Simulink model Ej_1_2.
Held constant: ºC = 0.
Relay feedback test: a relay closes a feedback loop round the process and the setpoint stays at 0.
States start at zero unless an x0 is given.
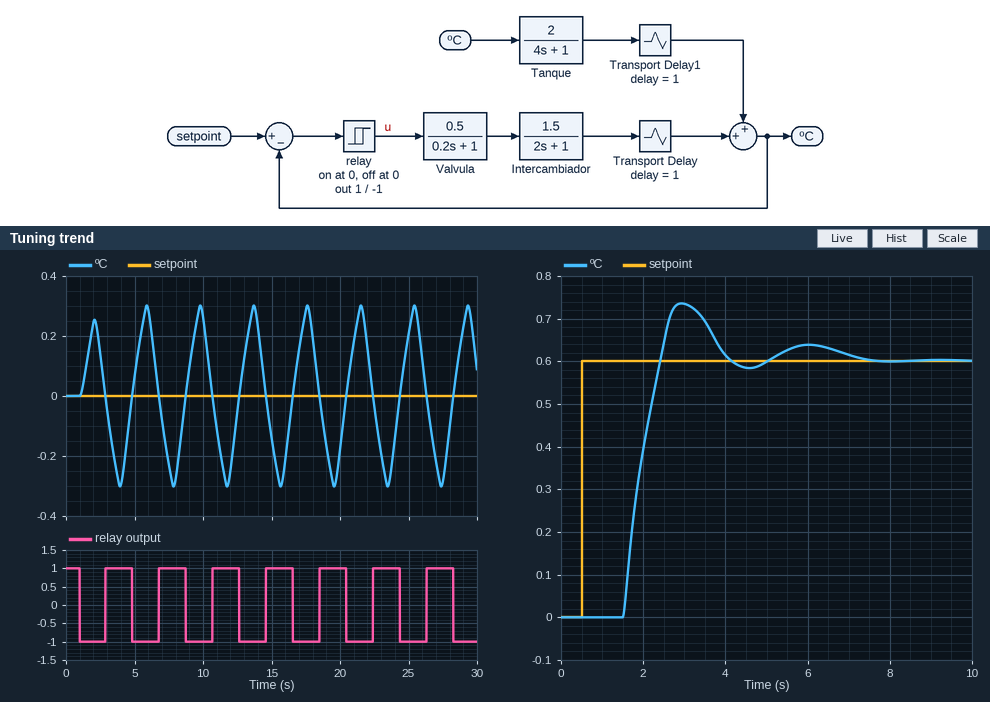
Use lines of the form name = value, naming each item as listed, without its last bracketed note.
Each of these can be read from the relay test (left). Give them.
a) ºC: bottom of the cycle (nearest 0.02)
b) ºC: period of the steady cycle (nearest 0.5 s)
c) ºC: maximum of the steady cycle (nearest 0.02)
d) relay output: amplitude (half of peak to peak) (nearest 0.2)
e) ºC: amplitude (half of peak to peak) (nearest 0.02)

ºC: bottom of the cycle = -0.30
ºC: period of the steady cycle = 4.0 s
ºC: maximum of the steady cycle = 0.30
relay output: amplitude (half of peak to peak) = 1.0
ºC: amplitude (half of peak to peak) = 0.30
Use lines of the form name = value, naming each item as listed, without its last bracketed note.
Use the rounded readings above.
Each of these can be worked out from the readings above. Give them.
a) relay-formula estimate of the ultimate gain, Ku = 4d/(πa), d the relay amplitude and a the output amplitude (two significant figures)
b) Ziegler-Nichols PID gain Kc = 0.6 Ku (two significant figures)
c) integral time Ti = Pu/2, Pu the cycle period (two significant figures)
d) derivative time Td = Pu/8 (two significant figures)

relay-formula estimate of the ultimate gain, Ku = 4d/(πa), d the relay amplitude and a the output amplitude = 4.2
Ziegler-Nichols PID gain Kc = 0.6 Ku = 2.5
integral time Ti = Pu/2, Pu the cycle period = 2.0 s
derivative time Td = Pu/8 = 0.50 s
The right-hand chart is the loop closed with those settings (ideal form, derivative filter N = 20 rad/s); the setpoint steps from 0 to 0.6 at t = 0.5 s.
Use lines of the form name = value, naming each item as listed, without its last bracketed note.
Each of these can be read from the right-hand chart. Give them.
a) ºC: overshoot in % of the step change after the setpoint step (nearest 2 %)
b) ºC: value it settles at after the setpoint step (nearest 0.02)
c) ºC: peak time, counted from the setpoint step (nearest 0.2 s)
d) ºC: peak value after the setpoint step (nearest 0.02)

ºC: overshoot in % of the step change after the setpoint step = 22 %
ºC: value it settles at after the setpoint step = 0.60
ºC: peak time, counted from the setpoint step = 2.4 s
ºC: peak value after the setpoint step = 0.74
